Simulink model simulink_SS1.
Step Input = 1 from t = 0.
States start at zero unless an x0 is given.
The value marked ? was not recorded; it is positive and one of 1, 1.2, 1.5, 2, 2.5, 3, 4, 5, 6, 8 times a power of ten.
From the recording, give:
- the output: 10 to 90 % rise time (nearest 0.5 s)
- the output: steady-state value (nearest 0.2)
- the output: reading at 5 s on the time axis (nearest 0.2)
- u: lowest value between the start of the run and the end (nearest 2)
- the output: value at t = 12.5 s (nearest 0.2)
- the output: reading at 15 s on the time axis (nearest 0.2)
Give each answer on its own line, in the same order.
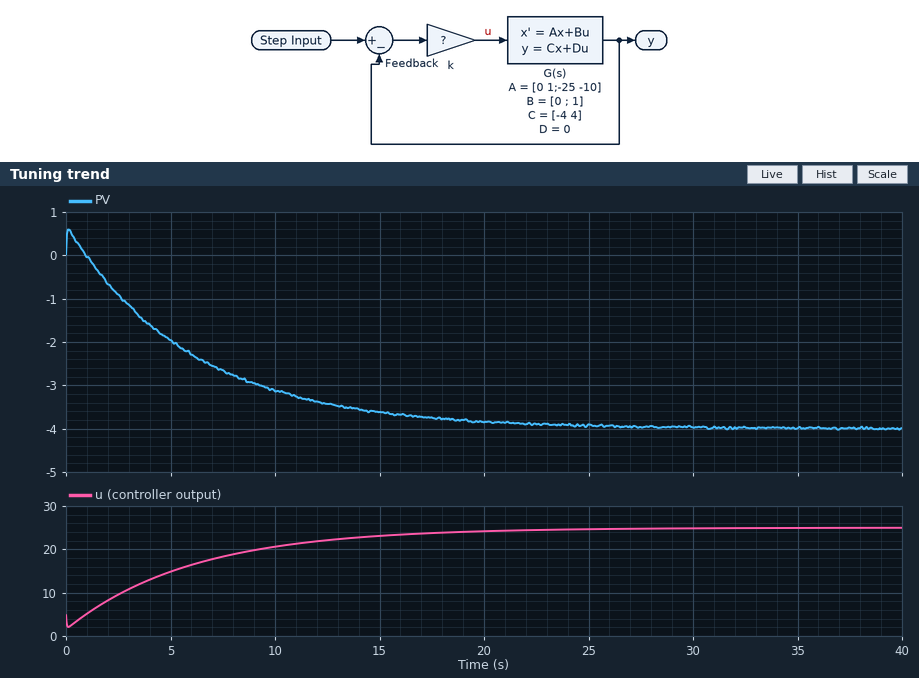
13.0 s
-4.0
-2.0
2
-3.4
-3.6
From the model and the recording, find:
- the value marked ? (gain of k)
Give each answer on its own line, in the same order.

5
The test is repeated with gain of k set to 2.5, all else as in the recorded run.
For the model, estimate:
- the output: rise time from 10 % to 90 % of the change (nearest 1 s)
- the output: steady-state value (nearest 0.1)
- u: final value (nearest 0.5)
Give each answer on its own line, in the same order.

3 s
-0.7
4.0
